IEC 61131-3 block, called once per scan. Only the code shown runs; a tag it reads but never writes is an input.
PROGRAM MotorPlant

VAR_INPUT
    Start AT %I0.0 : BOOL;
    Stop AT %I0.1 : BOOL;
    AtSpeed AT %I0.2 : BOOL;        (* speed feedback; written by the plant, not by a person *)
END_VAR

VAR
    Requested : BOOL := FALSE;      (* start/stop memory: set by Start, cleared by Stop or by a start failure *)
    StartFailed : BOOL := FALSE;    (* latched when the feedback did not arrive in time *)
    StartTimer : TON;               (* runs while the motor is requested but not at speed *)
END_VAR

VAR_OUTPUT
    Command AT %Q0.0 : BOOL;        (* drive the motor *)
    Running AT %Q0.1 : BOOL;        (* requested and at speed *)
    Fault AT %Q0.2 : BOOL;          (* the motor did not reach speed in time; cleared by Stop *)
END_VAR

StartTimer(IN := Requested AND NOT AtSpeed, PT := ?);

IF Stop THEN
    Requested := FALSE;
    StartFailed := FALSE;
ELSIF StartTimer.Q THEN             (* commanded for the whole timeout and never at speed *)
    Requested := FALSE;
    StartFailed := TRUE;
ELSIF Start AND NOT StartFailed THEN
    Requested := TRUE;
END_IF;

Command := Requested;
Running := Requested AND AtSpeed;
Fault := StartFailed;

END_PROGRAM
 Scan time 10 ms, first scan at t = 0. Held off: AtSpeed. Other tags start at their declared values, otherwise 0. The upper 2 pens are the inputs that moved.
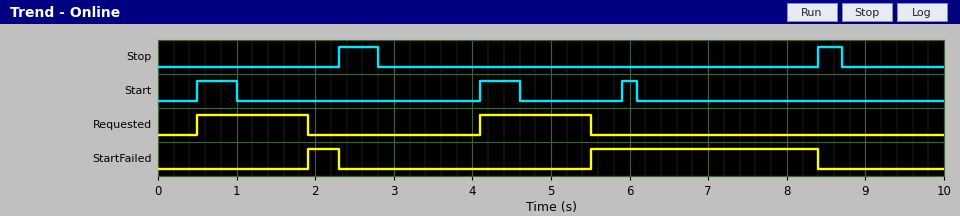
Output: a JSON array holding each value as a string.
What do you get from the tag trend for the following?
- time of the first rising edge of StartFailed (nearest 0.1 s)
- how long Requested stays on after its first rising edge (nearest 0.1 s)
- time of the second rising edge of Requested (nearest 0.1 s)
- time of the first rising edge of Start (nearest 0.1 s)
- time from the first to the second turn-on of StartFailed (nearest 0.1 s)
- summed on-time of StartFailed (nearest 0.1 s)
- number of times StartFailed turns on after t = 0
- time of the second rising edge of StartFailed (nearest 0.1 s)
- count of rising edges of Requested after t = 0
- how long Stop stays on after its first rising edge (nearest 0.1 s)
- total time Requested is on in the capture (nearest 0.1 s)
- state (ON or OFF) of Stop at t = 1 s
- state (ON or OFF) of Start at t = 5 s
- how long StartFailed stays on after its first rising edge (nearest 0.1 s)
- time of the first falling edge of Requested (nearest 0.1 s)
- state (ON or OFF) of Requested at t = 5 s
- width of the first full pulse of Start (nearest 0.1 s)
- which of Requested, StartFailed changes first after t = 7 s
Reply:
["1.9 s", "1.4 s", "4.1 s", "0.5 s", "3.6 s", "3.3 s", "2", "5.5 s", "2", "0.5 s", "2.8 s", "OFF", "OFF", "0.4 s", "1.9 s", "ON", "0.5 s", "StartFailed"]
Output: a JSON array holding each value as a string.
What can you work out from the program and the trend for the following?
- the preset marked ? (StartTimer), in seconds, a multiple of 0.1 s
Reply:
["1.4 s"]
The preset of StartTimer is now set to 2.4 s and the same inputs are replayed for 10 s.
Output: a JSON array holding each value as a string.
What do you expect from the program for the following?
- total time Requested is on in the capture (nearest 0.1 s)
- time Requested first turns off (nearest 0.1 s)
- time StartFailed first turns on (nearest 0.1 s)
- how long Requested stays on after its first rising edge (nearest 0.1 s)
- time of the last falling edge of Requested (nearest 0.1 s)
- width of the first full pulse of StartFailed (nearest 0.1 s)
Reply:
["4.2 s", "2.3 s", "6.5 s", "1.8 s", "6.5 s", "1.9 s"]
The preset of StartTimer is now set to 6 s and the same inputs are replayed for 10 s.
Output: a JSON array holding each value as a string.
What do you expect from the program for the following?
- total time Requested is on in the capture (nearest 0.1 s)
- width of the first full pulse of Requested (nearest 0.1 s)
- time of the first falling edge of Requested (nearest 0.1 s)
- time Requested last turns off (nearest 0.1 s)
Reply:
["6.1 s", "1.8 s", "2.3 s", "8.4 s"]
